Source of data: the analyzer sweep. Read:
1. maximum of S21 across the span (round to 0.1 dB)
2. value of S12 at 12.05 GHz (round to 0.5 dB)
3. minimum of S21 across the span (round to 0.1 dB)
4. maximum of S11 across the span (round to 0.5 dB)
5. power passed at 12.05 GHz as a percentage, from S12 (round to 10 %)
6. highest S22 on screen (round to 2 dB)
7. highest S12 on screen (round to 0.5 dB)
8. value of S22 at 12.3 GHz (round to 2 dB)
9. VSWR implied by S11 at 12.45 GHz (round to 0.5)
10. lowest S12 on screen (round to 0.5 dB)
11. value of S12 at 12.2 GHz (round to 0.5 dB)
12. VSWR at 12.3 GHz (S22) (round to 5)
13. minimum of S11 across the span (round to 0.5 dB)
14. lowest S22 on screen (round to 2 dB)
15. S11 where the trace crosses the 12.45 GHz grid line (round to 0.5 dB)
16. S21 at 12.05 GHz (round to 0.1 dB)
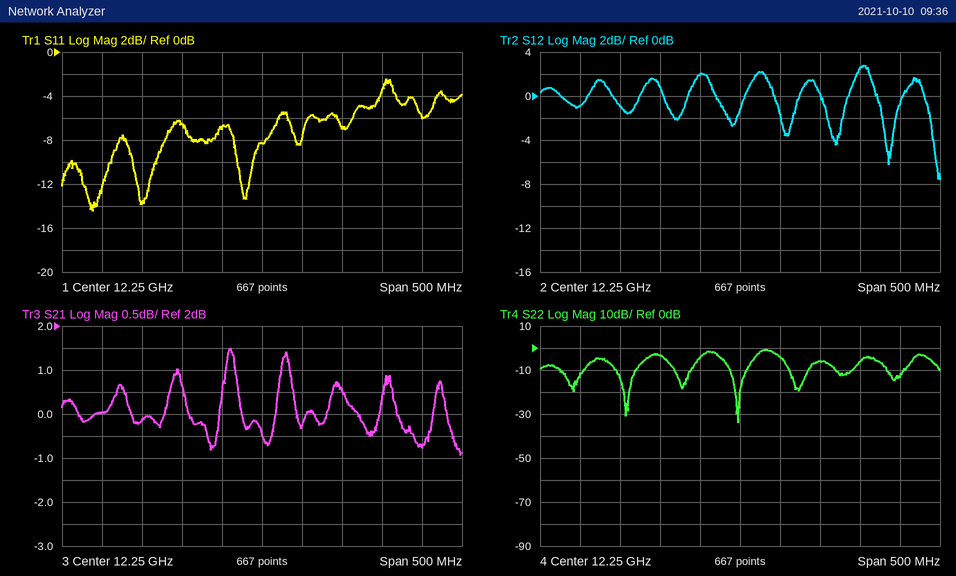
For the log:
1.5 dB
-1.0 dB
-0.9 dB
-2.5 dB
80 %
0 dB
3.0 dB
-4 dB
3.0
-7.5 dB
2.0 dB
5
-14.5 dB
-34 dB
-6.0 dB
0.0 dB
